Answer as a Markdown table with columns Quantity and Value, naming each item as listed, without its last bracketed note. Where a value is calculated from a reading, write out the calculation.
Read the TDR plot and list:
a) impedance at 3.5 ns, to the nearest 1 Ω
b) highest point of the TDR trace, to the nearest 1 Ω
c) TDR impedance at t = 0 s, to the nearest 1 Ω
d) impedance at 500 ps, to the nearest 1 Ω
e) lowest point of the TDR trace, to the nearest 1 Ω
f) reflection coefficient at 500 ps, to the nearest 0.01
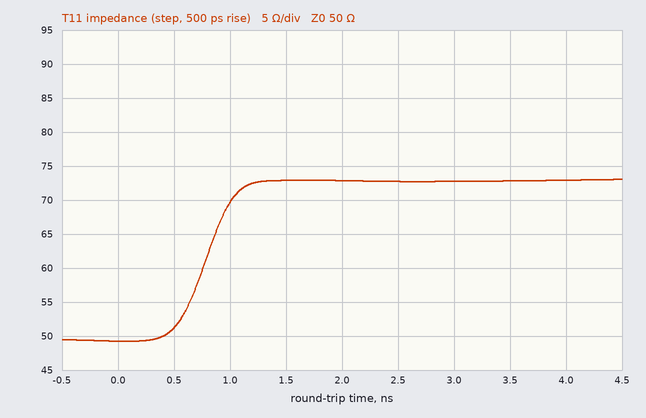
| Quantity | Value |
|---|---|
| impedance at 3.5 ns, to the nearest 1 Ω | 73 Ω |
| highest point of the TDR trace, to the nearest 1 Ω | 73 Ω |
| TDR impedance at t = 0 s, to the nearest 1 Ω | 49 Ω |
| impedance at 500 ps, to the nearest 1 Ω | 51 Ω |
| lowest point of the TDR trace, to the nearest 1 Ω | 49 Ω |
| reflection coefficient at 500 ps, to the nearest 0.01 | (51 − 50)/(51 + 50) ≈ +0.01 |
